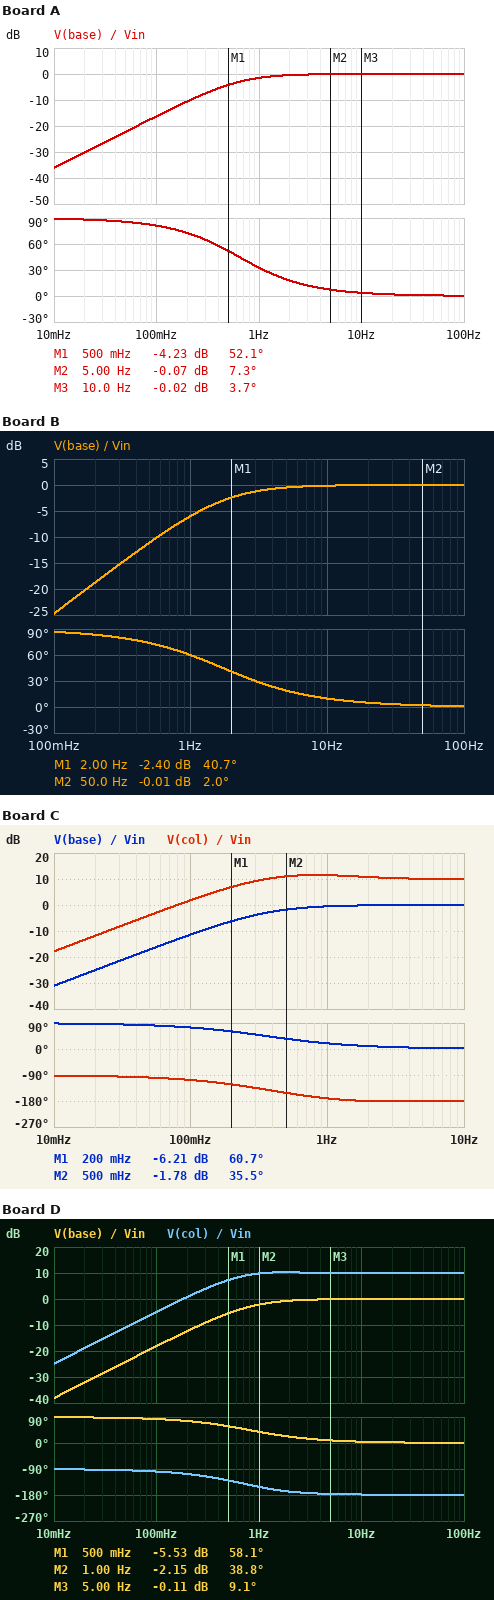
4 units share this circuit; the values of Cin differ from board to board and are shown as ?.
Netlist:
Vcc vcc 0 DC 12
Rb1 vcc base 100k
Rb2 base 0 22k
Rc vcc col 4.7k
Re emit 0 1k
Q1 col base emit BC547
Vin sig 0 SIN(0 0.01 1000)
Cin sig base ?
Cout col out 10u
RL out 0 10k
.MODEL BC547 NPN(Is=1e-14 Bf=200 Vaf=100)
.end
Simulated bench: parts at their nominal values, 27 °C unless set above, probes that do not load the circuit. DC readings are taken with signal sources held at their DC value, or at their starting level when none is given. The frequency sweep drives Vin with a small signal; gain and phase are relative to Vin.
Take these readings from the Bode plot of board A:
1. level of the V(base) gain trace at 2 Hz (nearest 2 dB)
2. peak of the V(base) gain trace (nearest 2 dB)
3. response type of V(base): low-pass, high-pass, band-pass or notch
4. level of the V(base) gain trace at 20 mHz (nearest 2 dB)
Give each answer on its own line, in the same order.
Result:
0 dB
0 dB
high-pass
-30 dB
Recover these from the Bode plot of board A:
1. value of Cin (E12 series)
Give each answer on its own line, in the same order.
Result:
15 µF
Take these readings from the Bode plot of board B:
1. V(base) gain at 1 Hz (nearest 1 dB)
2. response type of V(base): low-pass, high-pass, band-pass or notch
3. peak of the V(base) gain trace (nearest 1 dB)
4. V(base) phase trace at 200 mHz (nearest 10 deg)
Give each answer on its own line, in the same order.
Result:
-6 dB
high-pass
0 dB
80 deg
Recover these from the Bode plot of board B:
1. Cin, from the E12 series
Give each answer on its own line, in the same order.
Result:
5.6 µF
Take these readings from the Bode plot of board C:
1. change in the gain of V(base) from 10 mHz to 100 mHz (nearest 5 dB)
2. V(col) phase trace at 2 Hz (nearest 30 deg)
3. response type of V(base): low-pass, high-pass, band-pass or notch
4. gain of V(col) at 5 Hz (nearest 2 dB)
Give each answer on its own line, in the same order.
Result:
20 dB
-180 deg
high-pass
10 dB
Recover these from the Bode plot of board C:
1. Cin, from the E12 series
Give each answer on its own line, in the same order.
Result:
27 µF
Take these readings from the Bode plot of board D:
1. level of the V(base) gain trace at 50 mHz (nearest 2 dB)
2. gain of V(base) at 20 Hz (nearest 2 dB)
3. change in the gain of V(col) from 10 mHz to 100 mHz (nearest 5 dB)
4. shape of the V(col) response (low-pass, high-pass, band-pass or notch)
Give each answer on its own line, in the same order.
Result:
-24 dB
0 dB
20 dB
high-pass
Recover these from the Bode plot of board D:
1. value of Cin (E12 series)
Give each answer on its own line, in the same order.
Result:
12 µF
